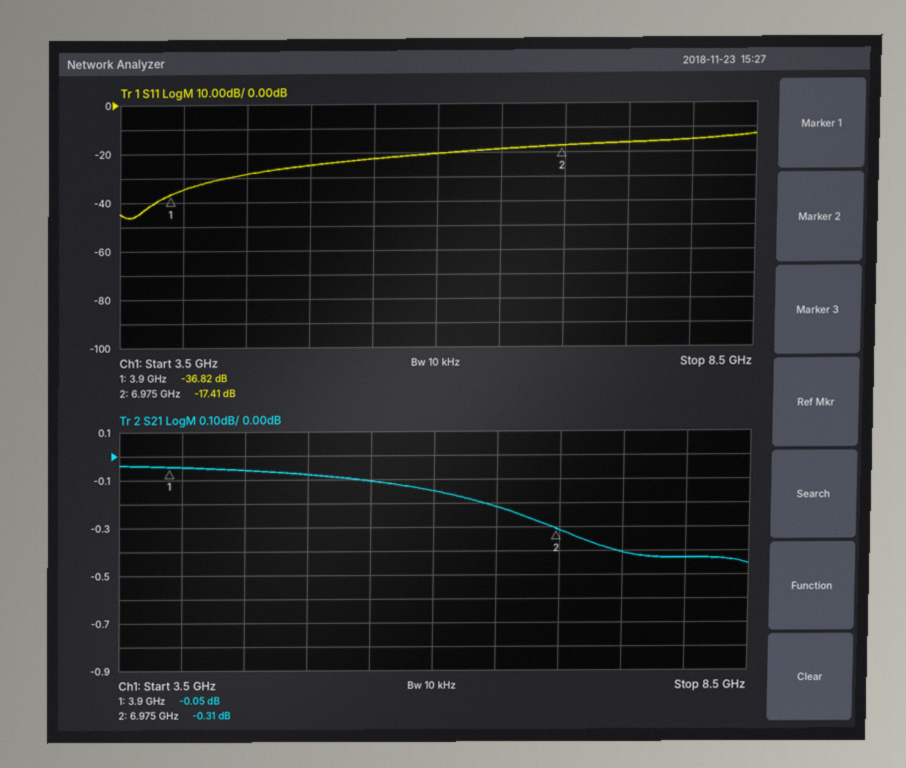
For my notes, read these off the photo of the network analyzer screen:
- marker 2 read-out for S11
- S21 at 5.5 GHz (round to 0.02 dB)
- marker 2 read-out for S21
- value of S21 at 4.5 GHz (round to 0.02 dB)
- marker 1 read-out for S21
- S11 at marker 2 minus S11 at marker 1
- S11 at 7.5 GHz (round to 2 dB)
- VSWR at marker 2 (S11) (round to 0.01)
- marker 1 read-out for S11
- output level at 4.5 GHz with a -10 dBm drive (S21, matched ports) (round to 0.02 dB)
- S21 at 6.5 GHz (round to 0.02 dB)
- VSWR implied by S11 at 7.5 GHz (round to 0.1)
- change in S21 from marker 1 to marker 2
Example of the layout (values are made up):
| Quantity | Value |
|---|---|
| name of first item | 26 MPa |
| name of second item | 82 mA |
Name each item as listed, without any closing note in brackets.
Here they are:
| Quantity | Value |
|---|---|
| marker 2 read-out for S11 | -17.41 dB |
| S21 at 5.5 GHz | -0.10 dB |
| marker 2 read-out for S21 | -0.31 dB |
| value of S21 at 4.5 GHz | -0.06 dB |
| marker 1 read-out for S21 | -0.05 dB |
| S11 at marker 2 minus S11 at marker 1 | 19.41 dB |
| S11 at 7.5 GHz | -16 dB |
| VSWR at marker 2 (S11) | 1.31 |
| marker 1 read-out for S11 | -36.82 dB |
| output level at 4.5 GHz with a -10 dBm drive (S21, matched ports) | -10.06 dBm |
| S21 at 6.5 GHz | -0.22 dB |
| VSWR implied by S11 at 7.5 GHz | 1.4 |
| change in S21 from marker 1 to marker 2 | -0.26 dB |
